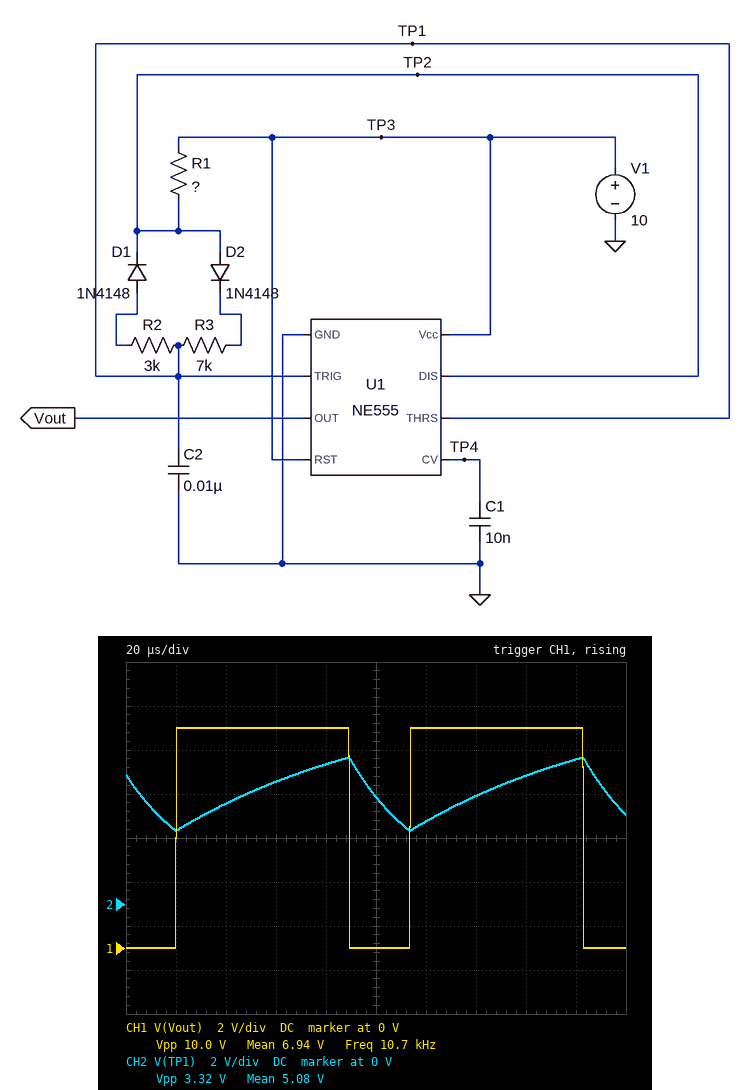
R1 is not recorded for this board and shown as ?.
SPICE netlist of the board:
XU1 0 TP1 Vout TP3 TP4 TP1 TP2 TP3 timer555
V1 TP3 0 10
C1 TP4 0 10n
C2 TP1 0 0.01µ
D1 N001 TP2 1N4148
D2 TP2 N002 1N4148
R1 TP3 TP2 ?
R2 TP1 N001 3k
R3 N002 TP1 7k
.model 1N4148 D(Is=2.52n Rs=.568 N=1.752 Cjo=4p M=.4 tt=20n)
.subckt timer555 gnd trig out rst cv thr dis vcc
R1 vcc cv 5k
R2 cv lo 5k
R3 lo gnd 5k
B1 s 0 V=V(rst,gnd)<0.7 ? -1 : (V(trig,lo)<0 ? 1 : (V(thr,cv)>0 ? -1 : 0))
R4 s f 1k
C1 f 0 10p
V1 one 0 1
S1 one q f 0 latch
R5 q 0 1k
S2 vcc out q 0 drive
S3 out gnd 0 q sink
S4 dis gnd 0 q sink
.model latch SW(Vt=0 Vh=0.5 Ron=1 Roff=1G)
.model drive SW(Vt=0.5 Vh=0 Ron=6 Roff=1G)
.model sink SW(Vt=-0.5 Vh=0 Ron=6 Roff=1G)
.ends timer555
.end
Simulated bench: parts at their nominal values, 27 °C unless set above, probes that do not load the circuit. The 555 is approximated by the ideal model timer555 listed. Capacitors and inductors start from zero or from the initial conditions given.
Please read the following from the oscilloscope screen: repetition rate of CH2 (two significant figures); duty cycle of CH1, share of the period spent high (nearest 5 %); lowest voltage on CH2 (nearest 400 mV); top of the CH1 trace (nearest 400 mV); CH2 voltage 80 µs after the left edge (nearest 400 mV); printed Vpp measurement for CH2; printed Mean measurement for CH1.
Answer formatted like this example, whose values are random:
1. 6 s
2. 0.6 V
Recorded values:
1. 11 kHz
2. 75 %
3. 3.2 V
4. 10.0 V
5. 6.4 V
6. 3.32 V
7. 6.94 V
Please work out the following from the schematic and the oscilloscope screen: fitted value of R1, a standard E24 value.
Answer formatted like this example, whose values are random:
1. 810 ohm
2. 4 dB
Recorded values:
1. 1.8 kΩ
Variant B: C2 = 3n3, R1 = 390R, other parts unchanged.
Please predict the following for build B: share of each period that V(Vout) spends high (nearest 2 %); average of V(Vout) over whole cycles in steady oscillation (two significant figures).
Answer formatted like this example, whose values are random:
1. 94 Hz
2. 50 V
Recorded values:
1. 70 %
2. 7.0 V
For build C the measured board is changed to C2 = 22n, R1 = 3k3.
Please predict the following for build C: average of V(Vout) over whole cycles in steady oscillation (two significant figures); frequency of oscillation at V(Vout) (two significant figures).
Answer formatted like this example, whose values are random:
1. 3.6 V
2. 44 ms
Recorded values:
1. 7.7 V
2. 4.3 kHz
